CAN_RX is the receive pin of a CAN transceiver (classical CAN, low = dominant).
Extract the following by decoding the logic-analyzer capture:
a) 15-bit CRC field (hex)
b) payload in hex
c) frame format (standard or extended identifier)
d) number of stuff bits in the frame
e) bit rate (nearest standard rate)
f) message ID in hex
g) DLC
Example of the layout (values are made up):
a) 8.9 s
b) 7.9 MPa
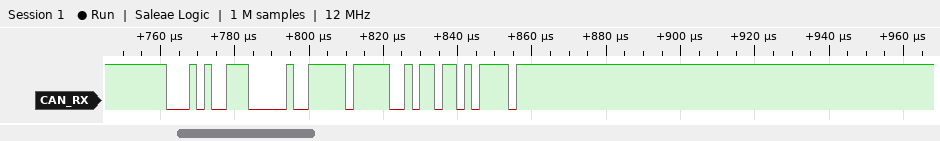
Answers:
a) 0x56D7
b) FF
c) standard
d) 3
e) 500 kbit/s
f) 0x14E
g) 1
